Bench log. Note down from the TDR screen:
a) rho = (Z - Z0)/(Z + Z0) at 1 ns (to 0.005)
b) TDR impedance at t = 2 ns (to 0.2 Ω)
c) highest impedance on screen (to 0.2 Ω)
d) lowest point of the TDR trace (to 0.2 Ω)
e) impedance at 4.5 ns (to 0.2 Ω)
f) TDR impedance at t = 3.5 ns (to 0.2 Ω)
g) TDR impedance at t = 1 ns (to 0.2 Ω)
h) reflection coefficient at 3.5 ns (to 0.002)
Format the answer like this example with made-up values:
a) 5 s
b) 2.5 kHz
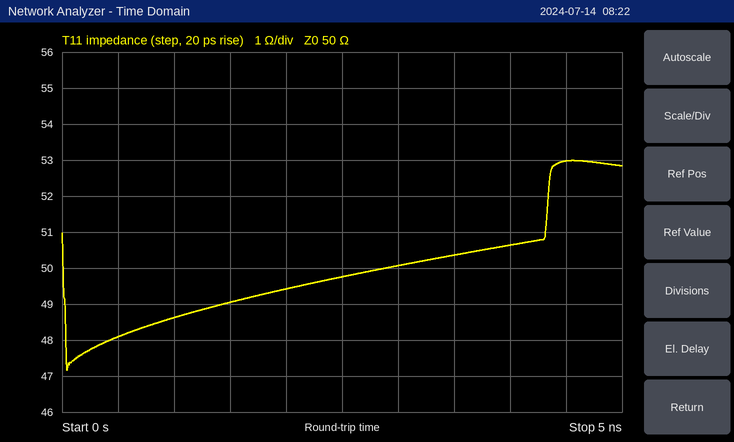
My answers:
a) -0.015
b) 49.4 Ω
c) 53.0 Ω
d) 47.2 Ω
e) 53.0 Ω
f) 50.4 Ω
g) 48.6 Ω
h) +0.004
